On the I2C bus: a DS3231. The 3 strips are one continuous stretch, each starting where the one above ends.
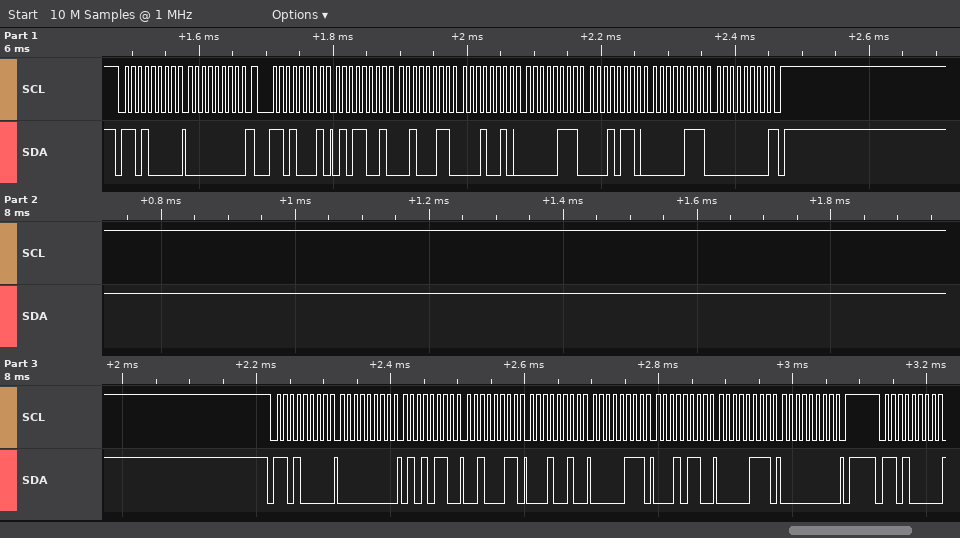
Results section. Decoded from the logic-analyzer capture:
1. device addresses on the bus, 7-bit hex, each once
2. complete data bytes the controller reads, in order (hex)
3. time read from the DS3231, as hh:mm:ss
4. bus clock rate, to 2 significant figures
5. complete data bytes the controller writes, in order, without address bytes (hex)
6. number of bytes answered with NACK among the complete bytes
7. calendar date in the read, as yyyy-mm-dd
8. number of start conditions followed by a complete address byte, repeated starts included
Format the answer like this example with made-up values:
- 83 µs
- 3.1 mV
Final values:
- 0x68
- 59 23 12 07 16 07 00
- 12:23:59
- 100 kHz
- 00 00 56 23 12 07 16 07 00
- 1
- 2000-07-16
- 4
